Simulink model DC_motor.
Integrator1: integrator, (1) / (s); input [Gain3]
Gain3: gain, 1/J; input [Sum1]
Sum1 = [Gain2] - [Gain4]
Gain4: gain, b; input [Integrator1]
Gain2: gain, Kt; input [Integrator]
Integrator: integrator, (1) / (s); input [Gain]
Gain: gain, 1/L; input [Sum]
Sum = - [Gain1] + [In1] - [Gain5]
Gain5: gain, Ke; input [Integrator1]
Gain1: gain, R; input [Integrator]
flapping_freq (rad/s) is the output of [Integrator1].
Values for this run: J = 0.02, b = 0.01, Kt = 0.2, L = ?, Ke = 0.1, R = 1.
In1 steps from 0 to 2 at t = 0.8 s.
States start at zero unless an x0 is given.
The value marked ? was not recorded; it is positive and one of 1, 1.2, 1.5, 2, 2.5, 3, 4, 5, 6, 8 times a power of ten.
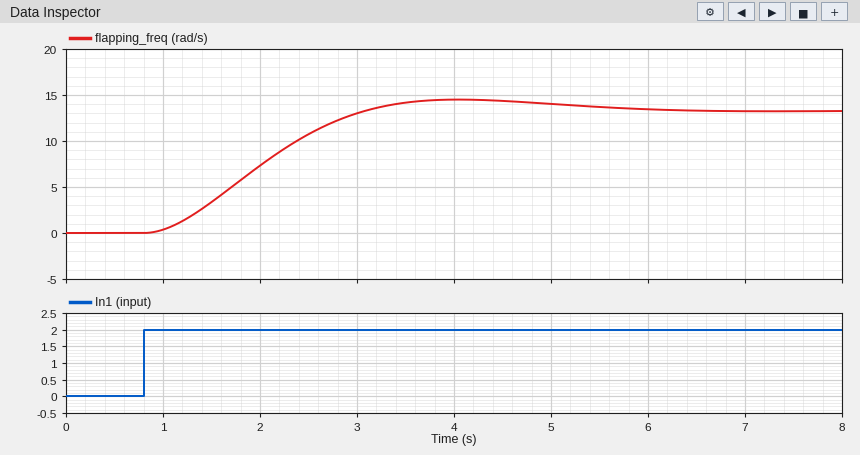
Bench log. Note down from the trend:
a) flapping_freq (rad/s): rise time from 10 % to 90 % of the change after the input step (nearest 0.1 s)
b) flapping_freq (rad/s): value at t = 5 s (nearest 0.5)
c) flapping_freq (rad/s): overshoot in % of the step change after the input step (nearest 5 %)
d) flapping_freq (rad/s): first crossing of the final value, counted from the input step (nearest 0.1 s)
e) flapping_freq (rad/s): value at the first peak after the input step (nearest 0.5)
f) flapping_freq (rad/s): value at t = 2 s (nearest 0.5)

1.5 s
14.0
10 %
2.3 s
14.5
7.5
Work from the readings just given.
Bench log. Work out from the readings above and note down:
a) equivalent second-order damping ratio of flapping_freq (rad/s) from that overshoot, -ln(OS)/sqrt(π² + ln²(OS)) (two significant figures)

0.59
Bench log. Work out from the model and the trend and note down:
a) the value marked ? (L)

1
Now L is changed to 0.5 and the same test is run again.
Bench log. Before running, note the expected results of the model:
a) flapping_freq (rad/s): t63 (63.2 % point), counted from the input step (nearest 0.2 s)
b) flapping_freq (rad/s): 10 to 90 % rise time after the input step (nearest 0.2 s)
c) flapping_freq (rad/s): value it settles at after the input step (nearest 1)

1.0 s
1.2 s
13
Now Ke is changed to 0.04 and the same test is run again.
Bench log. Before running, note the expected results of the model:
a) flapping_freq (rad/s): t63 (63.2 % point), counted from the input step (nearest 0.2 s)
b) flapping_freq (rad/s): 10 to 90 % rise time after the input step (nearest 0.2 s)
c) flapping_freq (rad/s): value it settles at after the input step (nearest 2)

2.0 s
2.6 s
22
